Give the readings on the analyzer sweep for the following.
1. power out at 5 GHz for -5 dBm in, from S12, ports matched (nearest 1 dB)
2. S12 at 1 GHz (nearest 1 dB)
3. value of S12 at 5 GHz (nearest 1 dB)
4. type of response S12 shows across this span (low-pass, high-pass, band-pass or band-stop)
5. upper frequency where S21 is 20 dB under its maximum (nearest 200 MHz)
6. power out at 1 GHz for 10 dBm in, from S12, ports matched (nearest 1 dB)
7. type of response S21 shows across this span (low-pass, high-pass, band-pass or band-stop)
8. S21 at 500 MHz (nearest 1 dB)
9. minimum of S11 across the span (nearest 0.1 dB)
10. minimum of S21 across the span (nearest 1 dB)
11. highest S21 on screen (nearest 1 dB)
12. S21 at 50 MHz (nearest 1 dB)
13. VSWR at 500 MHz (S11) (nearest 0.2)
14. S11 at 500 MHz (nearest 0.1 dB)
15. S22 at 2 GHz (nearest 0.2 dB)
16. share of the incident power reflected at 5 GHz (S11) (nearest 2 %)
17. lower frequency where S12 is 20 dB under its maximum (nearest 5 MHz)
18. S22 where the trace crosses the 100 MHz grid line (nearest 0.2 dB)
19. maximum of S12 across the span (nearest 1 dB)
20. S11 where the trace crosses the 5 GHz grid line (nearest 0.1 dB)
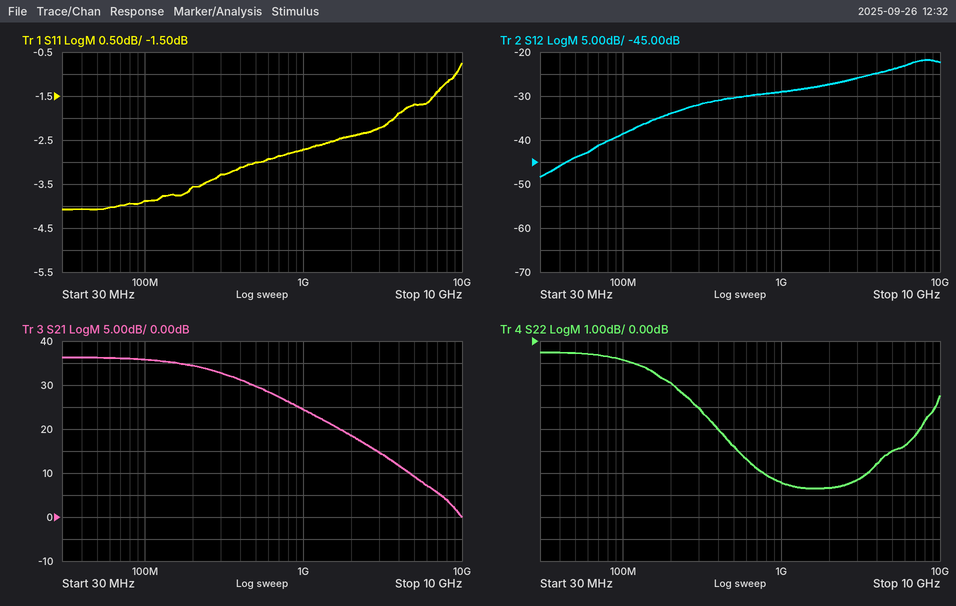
-29 dBm
-29 dB
-24 dB
high-pass
2.6 GHz
-19 dBm
low-pass
30 dB
-4.1 dB
0 dB
36 dB
36 dB
5.8
-3.0 dB
-6.6 dB
68 %
65 MHz
-0.8 dB
-22 dB
-1.7 dB
